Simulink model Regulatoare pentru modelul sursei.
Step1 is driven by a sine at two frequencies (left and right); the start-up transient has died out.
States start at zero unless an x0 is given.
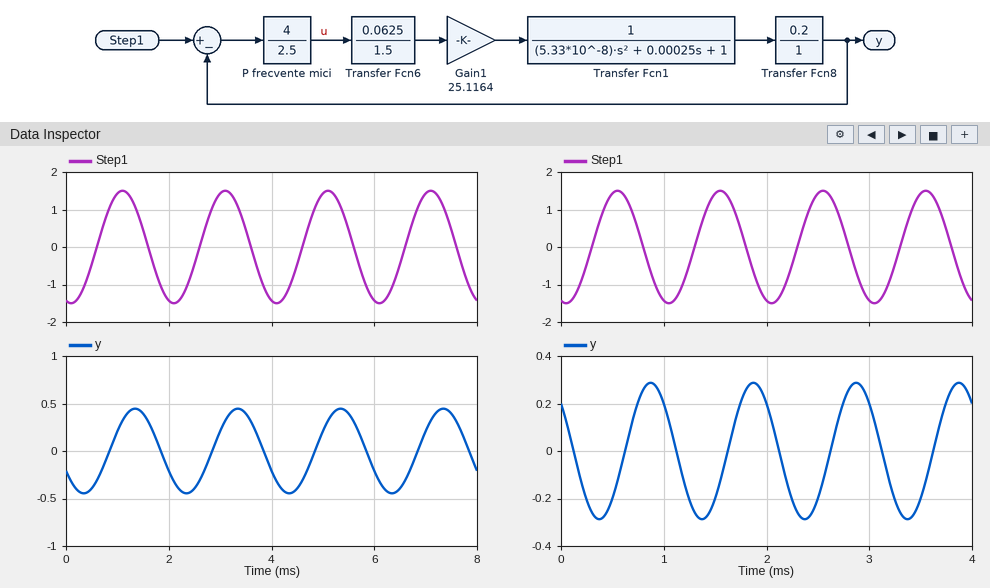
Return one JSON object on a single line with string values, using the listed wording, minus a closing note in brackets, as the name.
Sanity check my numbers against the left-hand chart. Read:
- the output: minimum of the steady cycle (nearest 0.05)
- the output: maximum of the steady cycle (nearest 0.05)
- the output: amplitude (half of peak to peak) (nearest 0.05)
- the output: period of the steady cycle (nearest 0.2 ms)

{"the output: minimum of the steady cycle": "-0.45", "the output: maximum of the steady cycle": "0.45", "the output: amplitude (half of peak to peak)": "0.45", "the output: period of the steady cycle": "2.0 ms"}
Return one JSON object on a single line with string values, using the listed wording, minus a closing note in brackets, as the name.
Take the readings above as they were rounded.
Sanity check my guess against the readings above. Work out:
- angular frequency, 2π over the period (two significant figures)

{"angular frequency, 2π over the period": "3.1 rad/ms"}
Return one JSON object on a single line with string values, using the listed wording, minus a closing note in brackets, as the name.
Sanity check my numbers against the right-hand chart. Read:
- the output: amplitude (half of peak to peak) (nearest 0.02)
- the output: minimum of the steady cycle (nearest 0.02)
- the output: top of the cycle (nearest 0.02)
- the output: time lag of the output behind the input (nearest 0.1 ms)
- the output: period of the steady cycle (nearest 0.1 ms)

{"the output: amplitude (half of peak to peak)": "0.28", "the output: minimum of the steady cycle": "-0.28", "the output: top of the cycle": "0.28", "the output: time lag of the output behind the input": "0.3 ms", "the output: period of the steady cycle": "1.0 ms"}
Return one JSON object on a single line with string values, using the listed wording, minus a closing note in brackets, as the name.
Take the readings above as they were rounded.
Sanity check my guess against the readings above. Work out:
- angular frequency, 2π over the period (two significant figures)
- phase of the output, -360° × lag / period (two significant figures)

{"angular frequency, 2π over the period": "6.3 rad/ms", "phase of the output, -360° × lag / period": "-110°"}
